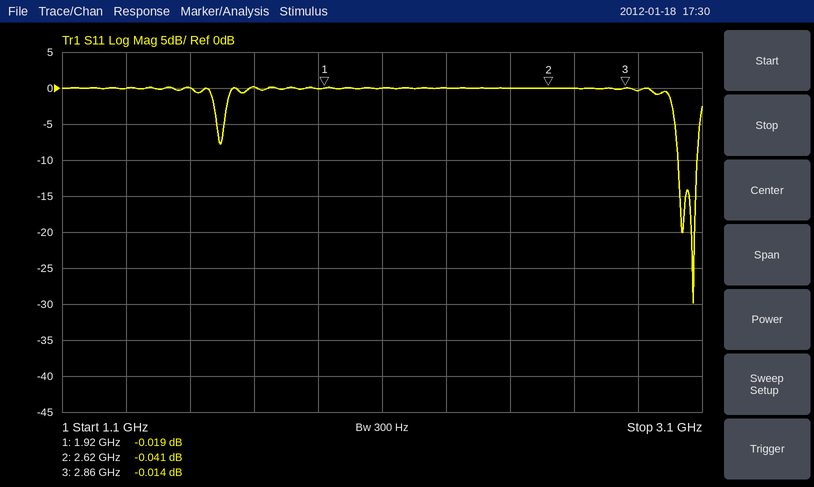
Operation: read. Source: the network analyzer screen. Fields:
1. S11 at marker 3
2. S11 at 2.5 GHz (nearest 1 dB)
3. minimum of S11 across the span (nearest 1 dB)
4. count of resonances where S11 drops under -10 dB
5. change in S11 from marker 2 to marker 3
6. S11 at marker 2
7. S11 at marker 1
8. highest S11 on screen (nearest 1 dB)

-0.014 dB
0 dB
-30 dB
2
0.027 dB
-0.041 dB
-0.019 dB
0 dB
